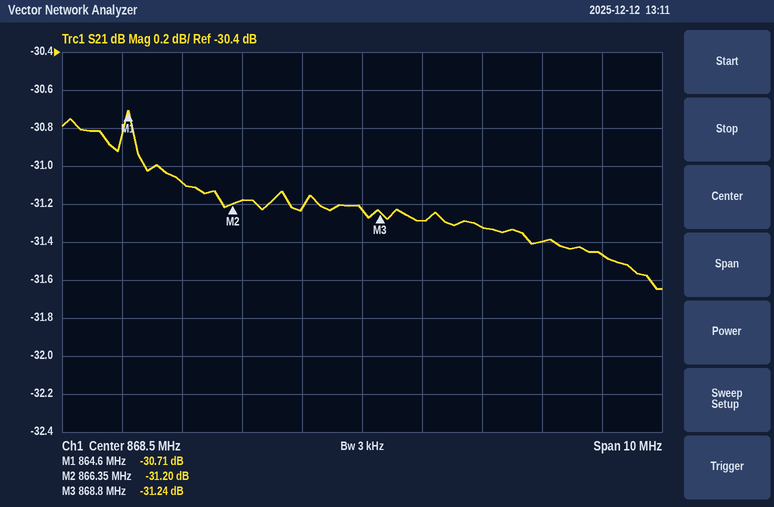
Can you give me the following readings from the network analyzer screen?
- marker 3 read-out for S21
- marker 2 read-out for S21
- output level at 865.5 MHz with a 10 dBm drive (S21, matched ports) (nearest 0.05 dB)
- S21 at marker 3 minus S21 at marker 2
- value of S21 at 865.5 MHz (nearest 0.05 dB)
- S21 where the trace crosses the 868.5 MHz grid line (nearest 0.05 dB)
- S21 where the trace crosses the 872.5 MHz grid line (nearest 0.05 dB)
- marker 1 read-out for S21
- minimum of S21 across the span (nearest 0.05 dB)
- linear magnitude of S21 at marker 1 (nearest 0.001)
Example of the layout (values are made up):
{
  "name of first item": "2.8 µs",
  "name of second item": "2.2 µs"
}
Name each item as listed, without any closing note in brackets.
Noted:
{
  "marker 3 read-out for S21": "-31.24 dB",
  "marker 2 read-out for S21": "-31.20 dB",
  "output level at 865.5 MHz with a 10 dBm drive (S21, matched ports)": "-21.10 dBm",
  "S21 at marker 3 minus S21 at marker 2": "-0.04 dB",
  "value of S21 at 865.5 MHz": "-31.10 dB",
  "S21 where the trace crosses the 868.5 MHz grid line": "-31.25 dB",
  "S21 where the trace crosses the 872.5 MHz grid line": "-31.45 dB",
  "marker 1 read-out for S21": "-30.71 dB",
  "minimum of S21 across the span": "-31.65 dB",
  "linear magnitude of S21 at marker 1": "0.029"
}
